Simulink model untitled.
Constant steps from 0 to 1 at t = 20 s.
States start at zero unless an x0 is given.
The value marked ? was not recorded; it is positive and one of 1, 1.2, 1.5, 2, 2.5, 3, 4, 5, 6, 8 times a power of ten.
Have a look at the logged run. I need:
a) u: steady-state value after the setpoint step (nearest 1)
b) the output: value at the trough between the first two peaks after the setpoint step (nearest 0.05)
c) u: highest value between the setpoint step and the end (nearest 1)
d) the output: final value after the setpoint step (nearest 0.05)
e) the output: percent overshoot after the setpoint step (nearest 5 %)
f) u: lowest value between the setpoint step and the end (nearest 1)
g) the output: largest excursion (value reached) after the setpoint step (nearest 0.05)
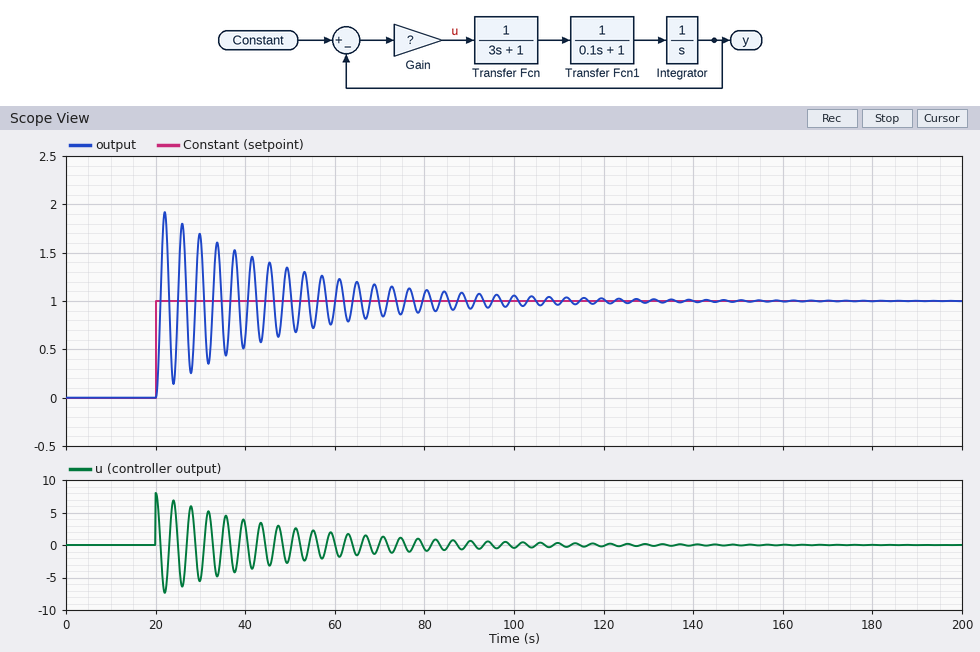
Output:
0
0.15
8
1.00
90 %
-7
1.90
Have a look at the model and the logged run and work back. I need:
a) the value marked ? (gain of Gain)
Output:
8
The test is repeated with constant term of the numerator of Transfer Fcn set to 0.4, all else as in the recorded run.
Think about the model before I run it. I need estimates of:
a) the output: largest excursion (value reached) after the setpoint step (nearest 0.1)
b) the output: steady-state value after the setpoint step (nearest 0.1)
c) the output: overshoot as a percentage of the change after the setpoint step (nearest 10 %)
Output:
1.7
1.0
70 %
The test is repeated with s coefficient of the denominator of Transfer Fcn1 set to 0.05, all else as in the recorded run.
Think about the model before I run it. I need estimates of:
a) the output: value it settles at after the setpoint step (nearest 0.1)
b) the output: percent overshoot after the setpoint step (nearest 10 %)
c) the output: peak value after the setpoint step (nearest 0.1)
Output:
1.0
80 %
1.8
